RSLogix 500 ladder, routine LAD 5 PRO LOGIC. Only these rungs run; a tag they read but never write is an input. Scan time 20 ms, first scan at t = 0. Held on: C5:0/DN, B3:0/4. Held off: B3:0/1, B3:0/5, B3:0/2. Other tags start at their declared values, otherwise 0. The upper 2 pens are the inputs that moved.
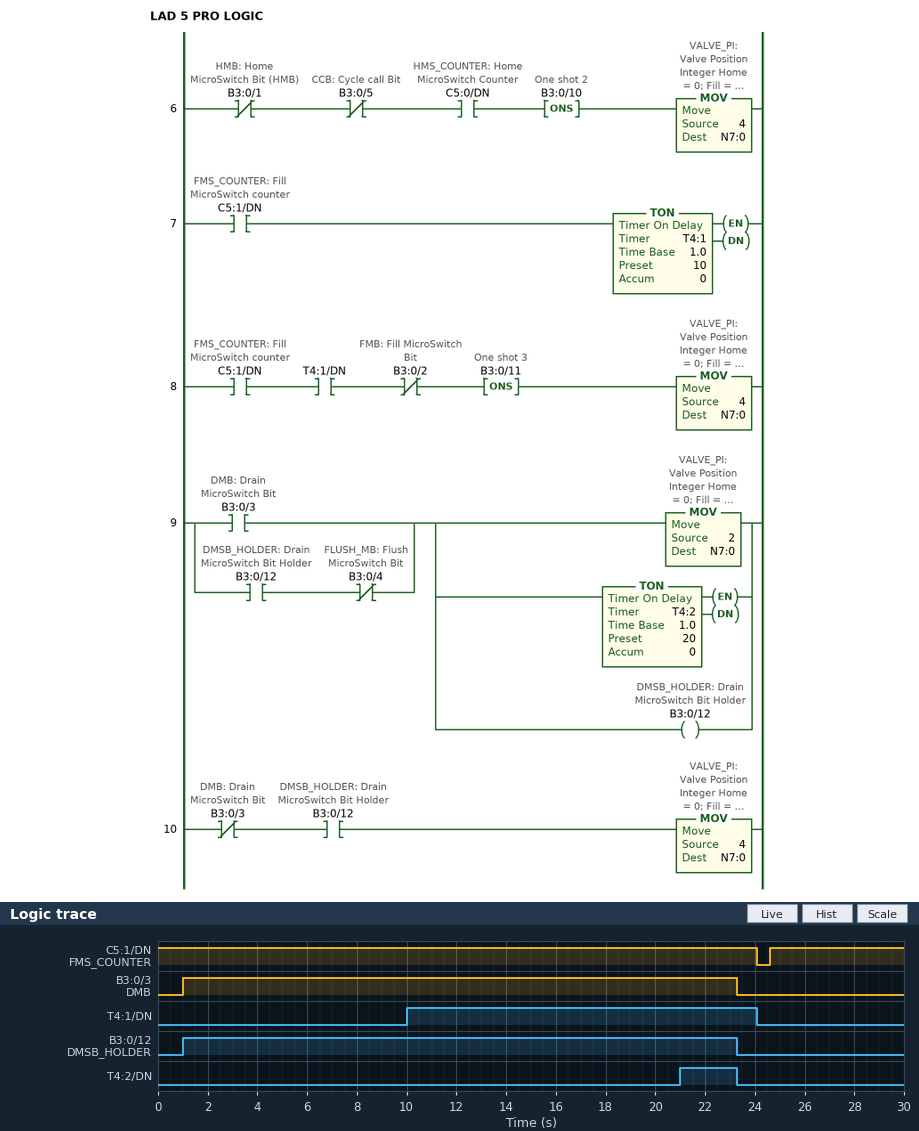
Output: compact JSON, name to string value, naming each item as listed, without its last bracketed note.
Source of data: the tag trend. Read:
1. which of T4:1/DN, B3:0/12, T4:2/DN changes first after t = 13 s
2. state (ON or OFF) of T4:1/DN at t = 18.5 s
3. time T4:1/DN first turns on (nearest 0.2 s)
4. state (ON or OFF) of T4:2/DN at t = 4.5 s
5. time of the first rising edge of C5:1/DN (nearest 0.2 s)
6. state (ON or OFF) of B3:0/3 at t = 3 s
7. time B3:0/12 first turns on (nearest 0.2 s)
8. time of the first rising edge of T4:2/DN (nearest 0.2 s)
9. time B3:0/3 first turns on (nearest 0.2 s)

{"which of T4:1/DN, B3:0/12, T4:2/DN changes first after t = 13 s": "T4:2/DN", "state (ON or OFF) of T4:1/DN at t = 18.5 s": "ON", "time T4:1/DN first turns on": "10.0 s", "state (ON or OFF) of T4:2/DN at t = 4.5 s": "OFF", "time of the first rising edge of C5:1/DN": "24.6 s", "state (ON or OFF) of B3:0/3 at t = 3 s": "ON", "time B3:0/12 first turns on": "1.0 s", "time of the first rising edge of T4:2/DN": "21.0 s", "time B3:0/3 first turns on": "1.0 s"}
